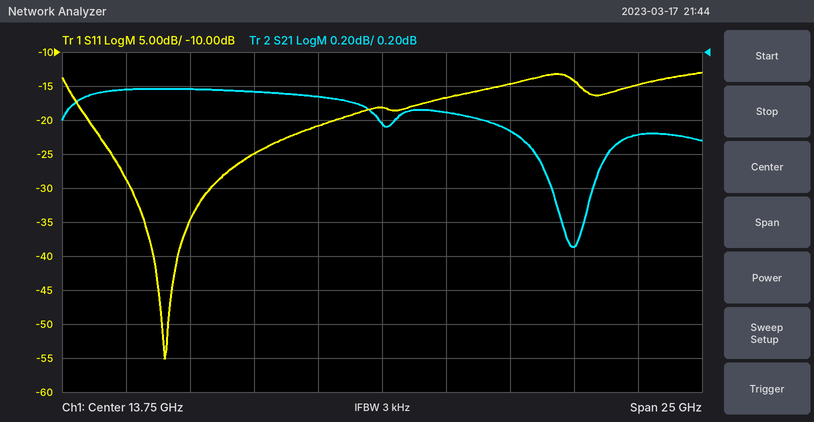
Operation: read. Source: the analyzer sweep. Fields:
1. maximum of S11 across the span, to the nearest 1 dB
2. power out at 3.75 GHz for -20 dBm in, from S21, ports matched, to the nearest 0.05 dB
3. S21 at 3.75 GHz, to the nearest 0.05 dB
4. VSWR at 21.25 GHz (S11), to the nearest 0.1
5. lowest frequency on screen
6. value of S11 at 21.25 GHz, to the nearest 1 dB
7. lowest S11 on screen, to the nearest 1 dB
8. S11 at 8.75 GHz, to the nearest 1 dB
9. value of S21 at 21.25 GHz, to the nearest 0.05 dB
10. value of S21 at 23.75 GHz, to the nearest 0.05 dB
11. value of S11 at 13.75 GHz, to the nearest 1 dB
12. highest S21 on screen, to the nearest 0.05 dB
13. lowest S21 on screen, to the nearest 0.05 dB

-13 dB
-20.00 dBm
0.00 dB
1.5
1.25 GHz
-14 dB
-55 dB
-25 dB
-0.95 dB
-0.30 dB
-18 dB
0.00 dB
-0.95 dB
